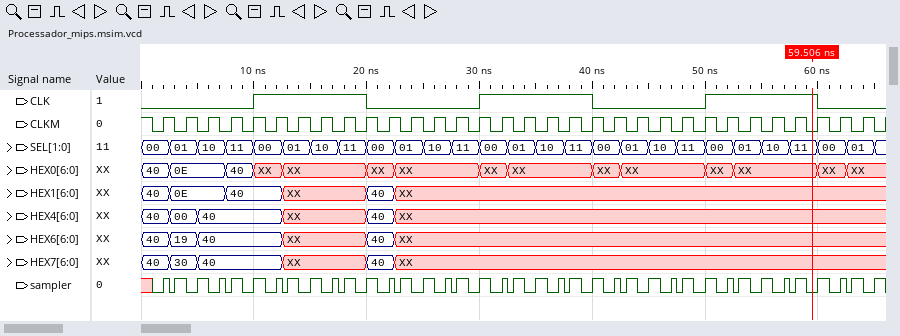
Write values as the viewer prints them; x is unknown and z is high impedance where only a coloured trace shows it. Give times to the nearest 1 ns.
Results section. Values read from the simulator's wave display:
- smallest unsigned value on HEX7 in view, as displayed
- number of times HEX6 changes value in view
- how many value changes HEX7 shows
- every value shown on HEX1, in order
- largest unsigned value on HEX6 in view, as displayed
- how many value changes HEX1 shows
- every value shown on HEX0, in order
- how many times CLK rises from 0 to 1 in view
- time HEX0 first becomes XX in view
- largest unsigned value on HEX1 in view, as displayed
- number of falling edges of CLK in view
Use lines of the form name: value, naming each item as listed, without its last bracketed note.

smallest unsigned value on HEX7 in view, as displayed: 30
number of times HEX6 changes value in view: 5
how many value changes HEX7 shows: 5
every value shown on HEX1, in order: 40, 0E, 40, XX, 40, XX
largest unsigned value on HEX6 in view, as displayed: 40
how many value changes HEX1 shows: 5
every value shown on HEX0, in order: 40, 0E, 40, XX, XX, XX, XX, XX, XX, XX, XX, XX, XX, XX, XX
how many times CLK rises from 0 to 1 in view: 3
time HEX0 first becomes XX in view: 10 ns
largest unsigned value on HEX1 in view, as displayed: 40
number of falling edges of CLK in view: 3
